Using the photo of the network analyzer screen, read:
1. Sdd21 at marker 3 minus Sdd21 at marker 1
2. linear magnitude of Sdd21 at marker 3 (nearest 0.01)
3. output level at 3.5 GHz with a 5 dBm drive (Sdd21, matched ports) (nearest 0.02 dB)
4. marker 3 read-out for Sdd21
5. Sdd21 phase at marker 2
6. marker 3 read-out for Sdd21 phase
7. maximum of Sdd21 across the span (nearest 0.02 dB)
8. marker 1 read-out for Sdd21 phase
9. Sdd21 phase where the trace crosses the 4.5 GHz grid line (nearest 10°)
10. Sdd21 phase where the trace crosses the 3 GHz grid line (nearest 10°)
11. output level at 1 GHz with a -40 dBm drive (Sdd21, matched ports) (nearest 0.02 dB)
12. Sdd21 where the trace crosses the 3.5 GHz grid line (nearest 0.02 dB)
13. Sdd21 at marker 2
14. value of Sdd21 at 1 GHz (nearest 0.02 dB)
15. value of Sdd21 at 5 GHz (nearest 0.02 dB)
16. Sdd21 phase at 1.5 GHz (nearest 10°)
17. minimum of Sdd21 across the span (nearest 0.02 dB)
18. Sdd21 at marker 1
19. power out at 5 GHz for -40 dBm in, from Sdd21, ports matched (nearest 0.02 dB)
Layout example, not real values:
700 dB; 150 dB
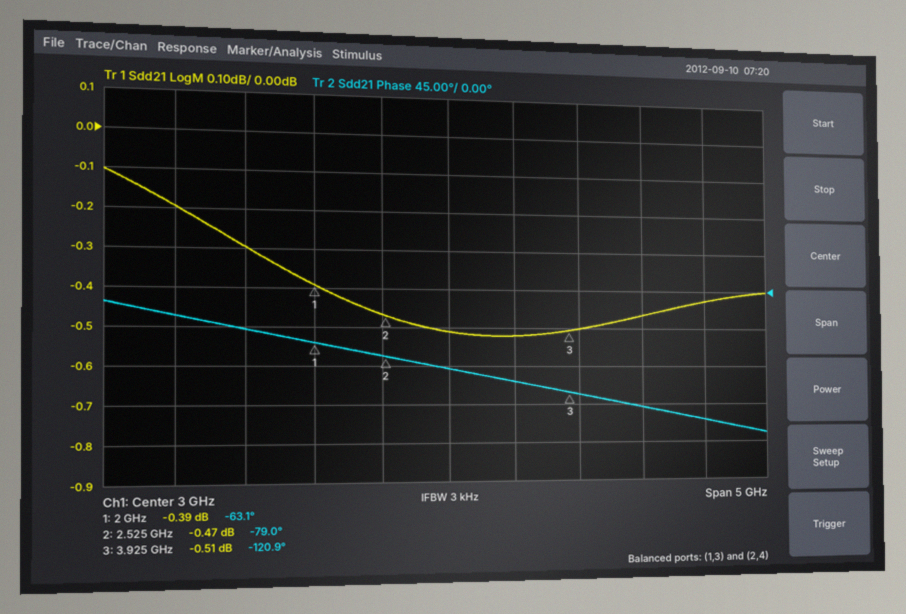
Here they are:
-0.12 dB; 0.94; 4.48 dBm; -0.51 dB; -79.0°; -120.9°; -0.10 dB; -63.1°; -140°; -90°; -40.20 dBm; -0.52 dB; -0.47 dB; -0.20 dB; -0.42 dB; -50°; -0.52 dB; -0.39 dB; -40.42 dBm
